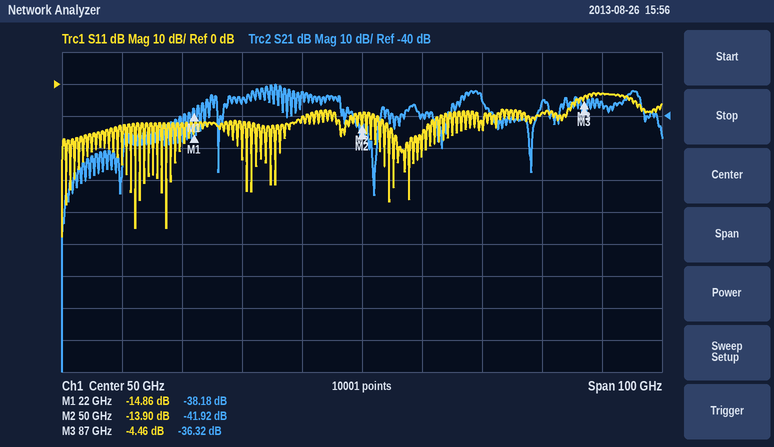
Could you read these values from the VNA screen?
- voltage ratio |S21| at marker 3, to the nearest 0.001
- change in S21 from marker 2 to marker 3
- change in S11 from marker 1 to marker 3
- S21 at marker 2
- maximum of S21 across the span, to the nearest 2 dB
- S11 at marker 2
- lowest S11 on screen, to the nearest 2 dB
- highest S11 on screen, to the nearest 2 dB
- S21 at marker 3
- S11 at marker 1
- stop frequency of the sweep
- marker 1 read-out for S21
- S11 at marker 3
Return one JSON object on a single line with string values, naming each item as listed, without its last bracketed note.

{"voltage ratio |S21| at marker 3, to the nearest 0.001": "0.015", "change in S21 from marker 2 to marker 3": "5.60 dB", "change in S11 from marker 1 to marker 3": "10.40 dB", "S21 at marker 2": "-41.92 dB", "maximum of S21 across the span, to the nearest 2 dB": "-30 dB", "S11 at marker 2": "-13.90 dB", "lowest S11 on screen, to the nearest 2 dB": "-48 dB", "highest S11 on screen, to the nearest 2 dB": "-2 dB", "S21 at marker 3": "-36.32 dB", "S11 at marker 1": "-14.86 dB", "stop frequency of the sweep": "100 GHz", "marker 1 read-out for S21": "-38.18 dB", "S11 at marker 3": "-4.46 dB"}
